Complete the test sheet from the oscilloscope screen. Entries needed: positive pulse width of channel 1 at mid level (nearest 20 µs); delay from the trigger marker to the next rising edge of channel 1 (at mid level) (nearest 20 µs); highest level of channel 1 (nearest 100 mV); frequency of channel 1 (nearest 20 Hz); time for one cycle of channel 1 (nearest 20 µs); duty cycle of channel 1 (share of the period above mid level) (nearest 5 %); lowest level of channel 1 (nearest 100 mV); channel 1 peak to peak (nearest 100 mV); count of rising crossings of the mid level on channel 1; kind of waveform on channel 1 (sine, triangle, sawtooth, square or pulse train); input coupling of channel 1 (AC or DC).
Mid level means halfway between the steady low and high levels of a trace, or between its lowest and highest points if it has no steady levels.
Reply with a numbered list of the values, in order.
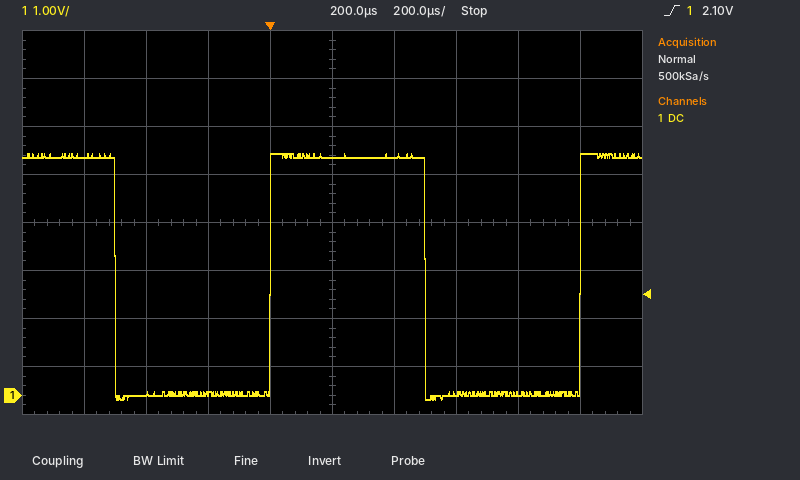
1. 500 µs
2. 1.00 ms
3. 5.0 V
4. 1.00 kHz
5. 1.00 ms
6. 50 %
7. -100 mV
8. 5.1 V
9. 2
10. square
11. DC
